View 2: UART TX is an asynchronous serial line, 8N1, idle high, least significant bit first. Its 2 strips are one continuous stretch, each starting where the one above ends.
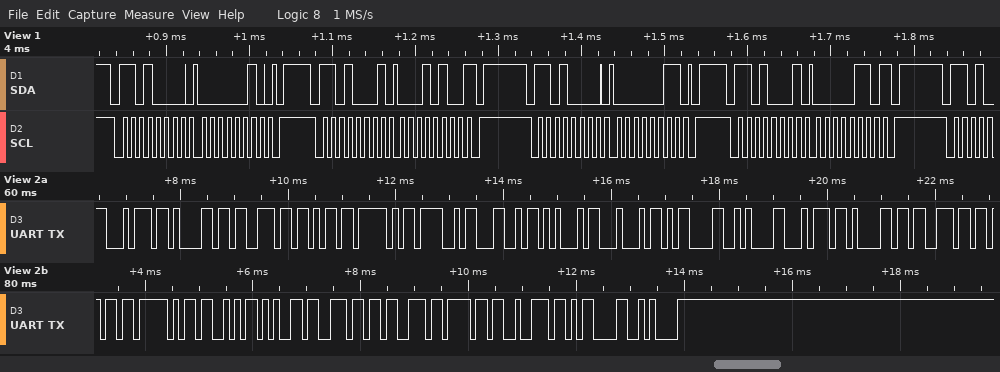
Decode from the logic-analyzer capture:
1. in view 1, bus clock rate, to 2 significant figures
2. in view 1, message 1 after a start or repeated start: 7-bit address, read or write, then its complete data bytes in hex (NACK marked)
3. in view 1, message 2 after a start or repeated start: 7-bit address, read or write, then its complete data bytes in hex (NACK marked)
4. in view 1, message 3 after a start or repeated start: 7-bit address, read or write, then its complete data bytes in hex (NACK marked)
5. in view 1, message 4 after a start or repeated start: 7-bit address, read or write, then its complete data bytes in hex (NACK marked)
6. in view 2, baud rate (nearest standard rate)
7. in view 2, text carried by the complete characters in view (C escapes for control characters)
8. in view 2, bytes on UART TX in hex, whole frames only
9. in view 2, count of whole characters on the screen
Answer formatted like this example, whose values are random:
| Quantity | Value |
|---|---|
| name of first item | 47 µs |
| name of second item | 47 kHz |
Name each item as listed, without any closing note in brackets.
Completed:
| Quantity | Value |
|---|---|
| in view 1, bus clock rate, to 2 significant figures | 100 kHz |
| in view 1, message 1 after a start or repeated start: 7-bit address, read or write, then its complete data bytes in hex | 0x68 write: 02 |
| in view 1, message 2 after a start or repeated start: 7-bit address, read or write, then its complete data bytes in hex | 0x68 read: 14 NACK |
| in view 1, message 3 after a start or repeated start: 7-bit address, read or write, then its complete data bytes in hex | 0x68 write: 03 |
| in view 1, message 4 after a start or repeated start: 7-bit address, read or write, then its complete data bytes in hex | 0x68 read: 06 NACK |
| in view 2, baud rate | 9600 baud |
| in view 2, text carried by the complete characters in view | "task_OLED\r\ntask_Sensor\r\n" |
| in view 2, bytes on UART TX in hex, whole frames only | 74 61 73 6B 5F 4F 4C 45 44 0D 0A 74 61 73 6B 5F 53 65 6E 73 6F 72 0D 0A |
| in view 2, count of whole characters on the screen | 24 |
